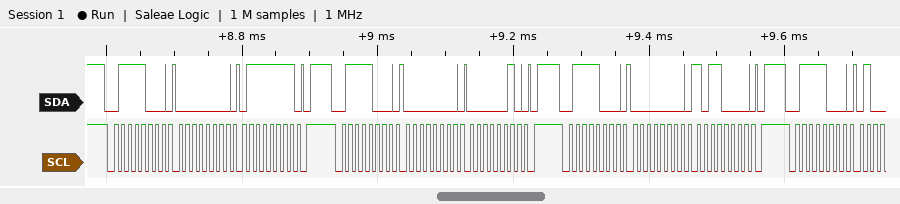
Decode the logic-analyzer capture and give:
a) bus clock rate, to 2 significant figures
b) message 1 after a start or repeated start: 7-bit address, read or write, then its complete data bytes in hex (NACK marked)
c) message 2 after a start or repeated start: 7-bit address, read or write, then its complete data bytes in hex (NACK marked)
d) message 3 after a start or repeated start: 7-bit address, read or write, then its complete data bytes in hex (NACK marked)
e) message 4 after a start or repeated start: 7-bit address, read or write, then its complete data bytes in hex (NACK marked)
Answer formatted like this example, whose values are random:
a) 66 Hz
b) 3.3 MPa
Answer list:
a) 100 kHz
b) 0x3C write: 00 7F
c) 0x3C write: 00 02
d) 0x3C write: 00 B0
e) 0x3C write
